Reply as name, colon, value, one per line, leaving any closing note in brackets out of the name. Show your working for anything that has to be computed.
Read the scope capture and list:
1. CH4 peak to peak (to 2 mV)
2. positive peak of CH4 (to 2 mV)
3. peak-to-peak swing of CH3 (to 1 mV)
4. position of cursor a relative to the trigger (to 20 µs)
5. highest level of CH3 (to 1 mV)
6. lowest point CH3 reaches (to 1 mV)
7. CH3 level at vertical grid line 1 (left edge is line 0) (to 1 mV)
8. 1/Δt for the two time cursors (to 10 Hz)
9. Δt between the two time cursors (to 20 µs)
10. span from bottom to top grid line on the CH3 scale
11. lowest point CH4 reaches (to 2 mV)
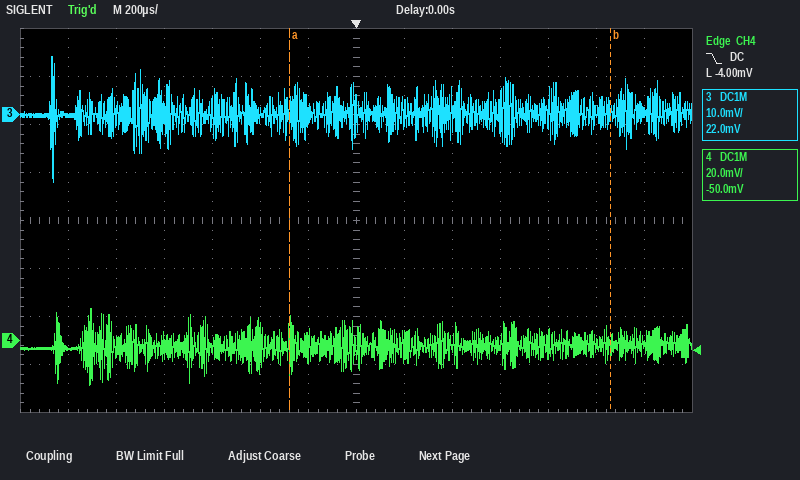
CH4 peak to peak: 14 mV − (-18 mV) = 32 mV
positive peak of CH4: 14 mV
peak-to-peak swing of CH3: 12 mV − (-14 mV) = 26 mV
position of cursor a relative to the trigger: -280 µs
highest level of CH3: 12 mV
lowest point CH3 reaches: -14 mV
CH3 level at vertical grid line 1 (left edge is line 0): 0 mV
1/Δt for the two time cursors: 1 / 1.34 ms ≈ 750 Hz
Δt between the two time cursors: 1.34 ms
span from bottom to top grid line on the CH3 scale: 80 mV
lowest point CH4 reaches: -18 mV
